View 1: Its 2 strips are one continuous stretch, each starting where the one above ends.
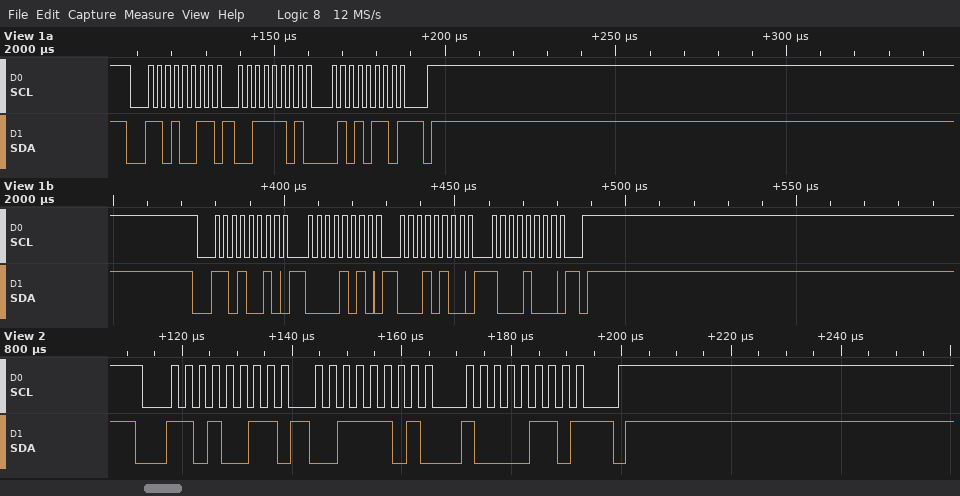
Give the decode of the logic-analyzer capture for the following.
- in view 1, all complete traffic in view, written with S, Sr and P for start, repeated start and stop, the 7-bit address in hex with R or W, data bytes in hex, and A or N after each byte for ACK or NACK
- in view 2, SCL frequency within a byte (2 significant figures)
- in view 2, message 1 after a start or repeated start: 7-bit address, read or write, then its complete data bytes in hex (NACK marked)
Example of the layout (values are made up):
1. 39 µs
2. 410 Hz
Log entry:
1. S 69R A 3D A 56 N P S 69W A 0A A 14 A 88 A P
2. 400 kHz
3. 0x69 read: 3D 86 NACK
